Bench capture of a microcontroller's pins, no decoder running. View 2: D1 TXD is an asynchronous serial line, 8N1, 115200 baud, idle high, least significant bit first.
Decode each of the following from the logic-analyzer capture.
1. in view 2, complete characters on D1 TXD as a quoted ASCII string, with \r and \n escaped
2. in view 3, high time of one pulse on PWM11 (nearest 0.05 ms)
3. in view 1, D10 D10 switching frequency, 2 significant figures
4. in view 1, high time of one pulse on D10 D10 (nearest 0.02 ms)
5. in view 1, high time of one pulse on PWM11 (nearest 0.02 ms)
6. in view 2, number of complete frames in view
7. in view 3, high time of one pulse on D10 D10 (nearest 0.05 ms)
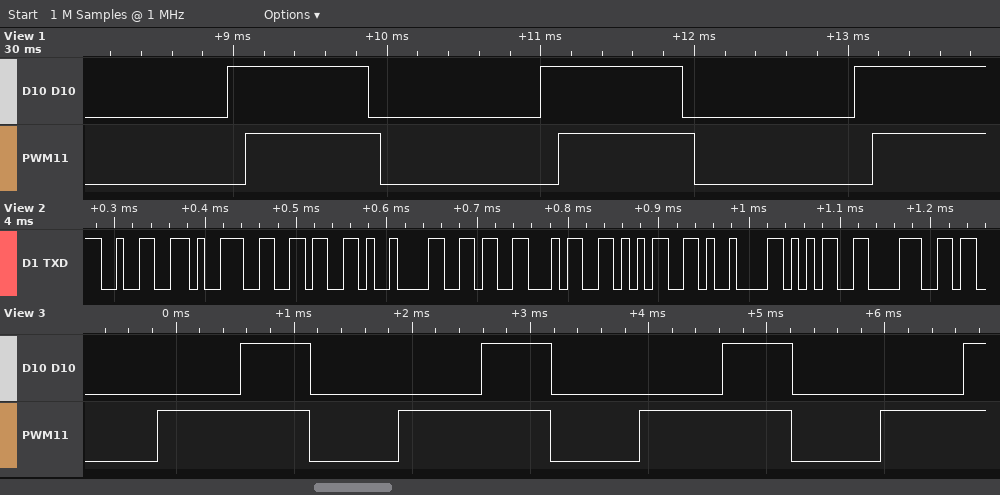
"296\t645\t58"
1.30 ms
490 Hz
0.92 ms
0.88 ms
10
0.60 ms
